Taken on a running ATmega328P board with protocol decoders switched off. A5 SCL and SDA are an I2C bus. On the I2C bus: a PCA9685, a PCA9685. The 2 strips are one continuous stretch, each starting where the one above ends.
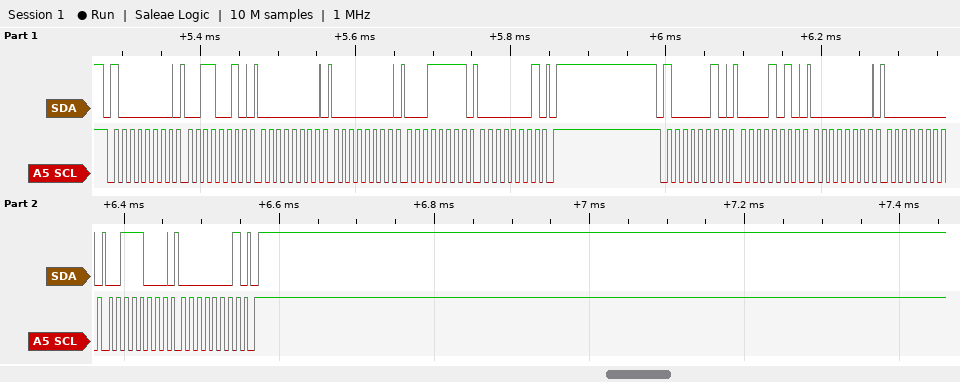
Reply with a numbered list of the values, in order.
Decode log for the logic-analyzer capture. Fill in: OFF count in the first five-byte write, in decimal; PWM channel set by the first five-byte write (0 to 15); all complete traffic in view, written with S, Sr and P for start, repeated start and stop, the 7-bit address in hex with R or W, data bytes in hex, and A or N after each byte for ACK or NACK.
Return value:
1. 287
2. 11
3. S 40W A 32 A 00 A 00 A 1F A 01 A P S 41W A 0A A 00 A 00 A 38 A 01 A P
